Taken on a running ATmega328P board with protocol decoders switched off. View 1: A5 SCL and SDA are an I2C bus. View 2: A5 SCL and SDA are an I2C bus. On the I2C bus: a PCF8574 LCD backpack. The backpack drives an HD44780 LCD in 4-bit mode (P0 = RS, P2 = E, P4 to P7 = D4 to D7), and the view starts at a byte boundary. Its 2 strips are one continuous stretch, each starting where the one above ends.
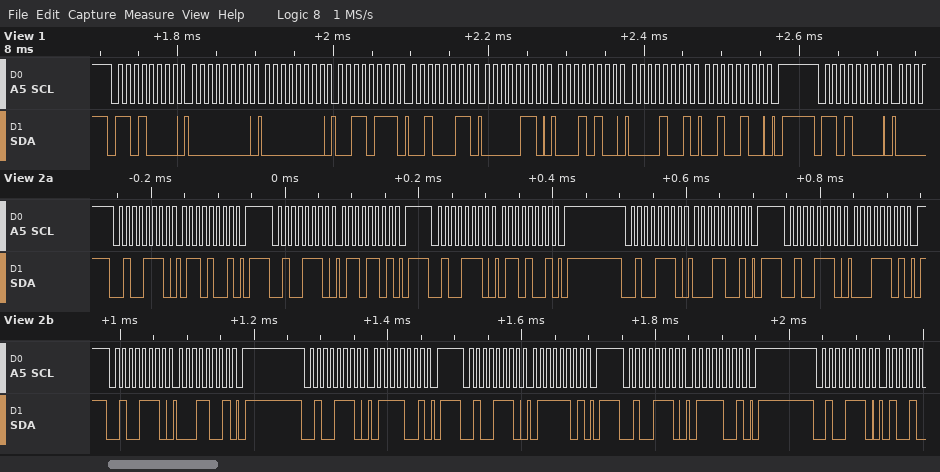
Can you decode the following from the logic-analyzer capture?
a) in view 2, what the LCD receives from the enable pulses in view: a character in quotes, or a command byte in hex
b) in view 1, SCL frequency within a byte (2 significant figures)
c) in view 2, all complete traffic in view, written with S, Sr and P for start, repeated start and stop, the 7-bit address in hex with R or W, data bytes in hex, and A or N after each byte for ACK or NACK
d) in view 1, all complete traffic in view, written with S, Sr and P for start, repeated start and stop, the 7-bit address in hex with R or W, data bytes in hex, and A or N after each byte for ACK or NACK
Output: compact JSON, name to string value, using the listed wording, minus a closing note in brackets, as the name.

{"in view 2, what the LCD receives from the enable pulses in view: a character in quotes, or a command byte in hex": "'a'", "in view 1, SCL frequency within a byte": "100 kHz", "in view 2, all complete traffic in view, written with S, Sr and P for start, repeated start and stop, the 7-bit address in hex with R or W, data bytes in hex, and A or N after each byte for ACK or NACK": "S 27W A 69 A P S 27W A 6D A P S 27W A 69 A P S 27W A 19 A P S 27W A 1D A P S 27W A 19 A P S 27W A 79 A P S 27W A 7D A P S 27W A 79 A P S 27W A", "in view 1, all complete traffic in view, written with S, Sr and P for start, repeated start and stop, the 7-bit address in hex with R or W, data bytes in hex, and A or N after each byte for ACK or NACK": "S 68W A 00 A 00 A 37 A 23 A 06 A 14 A 09 A 24 A P S 68W A"}
